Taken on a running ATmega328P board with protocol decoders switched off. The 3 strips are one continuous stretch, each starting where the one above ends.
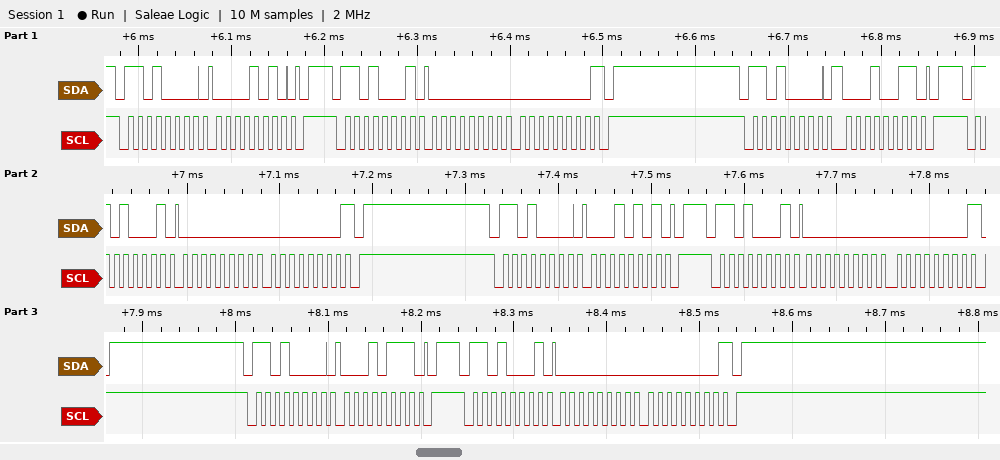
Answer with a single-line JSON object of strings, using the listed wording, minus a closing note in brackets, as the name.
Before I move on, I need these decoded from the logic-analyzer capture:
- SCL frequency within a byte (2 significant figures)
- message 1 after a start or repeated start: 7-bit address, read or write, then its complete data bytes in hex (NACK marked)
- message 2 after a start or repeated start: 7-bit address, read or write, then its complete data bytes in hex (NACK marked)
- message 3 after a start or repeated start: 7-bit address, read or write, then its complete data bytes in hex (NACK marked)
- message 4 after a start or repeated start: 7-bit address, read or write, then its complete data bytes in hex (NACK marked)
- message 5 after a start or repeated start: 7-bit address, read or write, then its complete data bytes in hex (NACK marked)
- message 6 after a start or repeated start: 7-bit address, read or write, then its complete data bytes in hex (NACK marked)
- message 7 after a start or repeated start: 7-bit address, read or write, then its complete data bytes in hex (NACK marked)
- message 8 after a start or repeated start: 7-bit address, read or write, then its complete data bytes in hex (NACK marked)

{"SCL frequency within a byte": "100 kHz", "message 1 after a start or repeated start: 7-bit address, read or write, then its complete data bytes in hex": "0x68 write: 0A", "message 2 after a start or repeated start: 7-bit address, read or write, then its complete data bytes in hex": "0x68 read: 00 00 NACK", "message 3 after a start or repeated start: 7-bit address, read or write, then its complete data bytes in hex": "0x68 write: 13", "message 4 after a start or repeated start: 7-bit address, read or write, then its complete data bytes in hex": "0x68 read: 00 00 NACK", "message 5 after a start or repeated start: 7-bit address, read or write, then its complete data bytes in hex": "0x68 write: 15", "message 6 after a start or repeated start: 7-bit address, read or write, then its complete data bytes in hex": "0x68 read: 00 00 NACK", "message 7 after a start or repeated start: 7-bit address, read or write, then its complete data bytes in hex": "0x68 write: 17", "message 8 after a start or repeated start: 7-bit address, read or write, then its complete data bytes in hex": "0x68 read: 00 00 NACK"}
